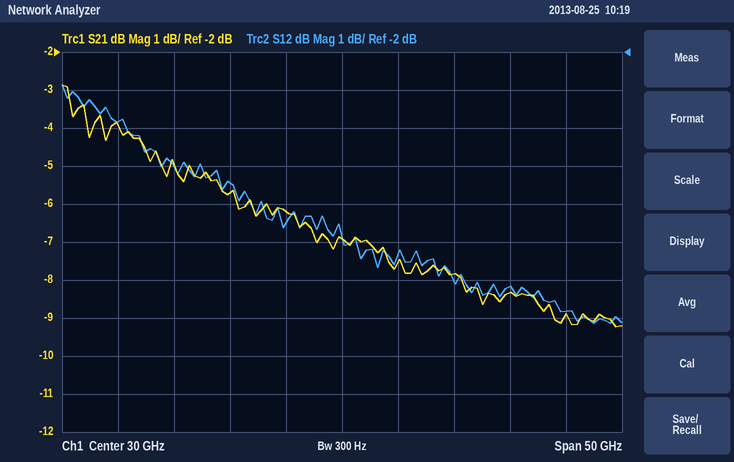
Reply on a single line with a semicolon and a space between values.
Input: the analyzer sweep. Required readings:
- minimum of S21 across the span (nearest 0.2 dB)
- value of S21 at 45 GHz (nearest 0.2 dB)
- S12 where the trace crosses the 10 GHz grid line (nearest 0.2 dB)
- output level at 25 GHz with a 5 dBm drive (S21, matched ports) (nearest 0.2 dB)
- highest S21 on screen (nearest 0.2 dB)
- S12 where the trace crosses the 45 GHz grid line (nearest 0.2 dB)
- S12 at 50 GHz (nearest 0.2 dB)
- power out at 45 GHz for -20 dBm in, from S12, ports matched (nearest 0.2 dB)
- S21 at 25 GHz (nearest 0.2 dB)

-9.2 dB; -8.4 dB; -3.8 dB; -1.2 dBm; -2.8 dB; -8.2 dB; -8.8 dB; -28.2 dBm; -6.2 dB
